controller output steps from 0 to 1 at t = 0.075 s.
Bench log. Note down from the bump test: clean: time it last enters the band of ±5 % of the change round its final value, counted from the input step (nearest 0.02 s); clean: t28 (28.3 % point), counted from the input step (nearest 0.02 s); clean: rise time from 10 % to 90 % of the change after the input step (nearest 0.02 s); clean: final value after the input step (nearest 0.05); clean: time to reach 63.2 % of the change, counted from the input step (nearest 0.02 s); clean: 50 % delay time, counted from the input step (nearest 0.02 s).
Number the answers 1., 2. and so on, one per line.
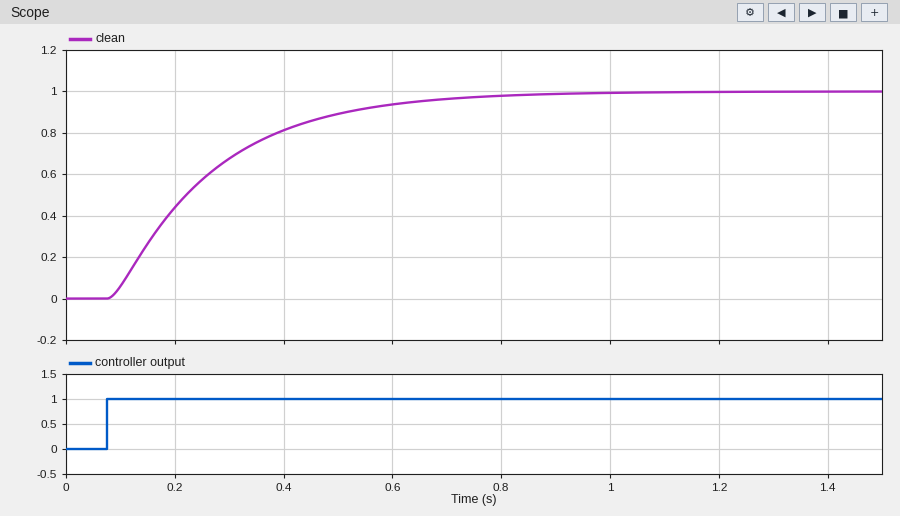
1. 0.56 s
2. 0.08 s
3. 0.40 s
4. 1.00
5. 0.20 s
6. 0.14 s
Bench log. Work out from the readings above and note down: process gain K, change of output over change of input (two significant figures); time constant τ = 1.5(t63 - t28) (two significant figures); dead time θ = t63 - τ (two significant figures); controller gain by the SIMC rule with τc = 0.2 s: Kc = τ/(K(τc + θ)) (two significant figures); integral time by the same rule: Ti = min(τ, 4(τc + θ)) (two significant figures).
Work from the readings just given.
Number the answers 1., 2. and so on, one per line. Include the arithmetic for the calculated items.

1. (1 - 0) / 1 = 1.0
2. 1.5 × (0.2 - 0.08) = 0.18 s
3. 0.2 - 0.18 = 0.020 s
4. 0.18 / (1 × (0.2 + 0.02)) = 0.82
5. min(0.18, 4 × (0.2 + 0.02)) = 0.18 s
